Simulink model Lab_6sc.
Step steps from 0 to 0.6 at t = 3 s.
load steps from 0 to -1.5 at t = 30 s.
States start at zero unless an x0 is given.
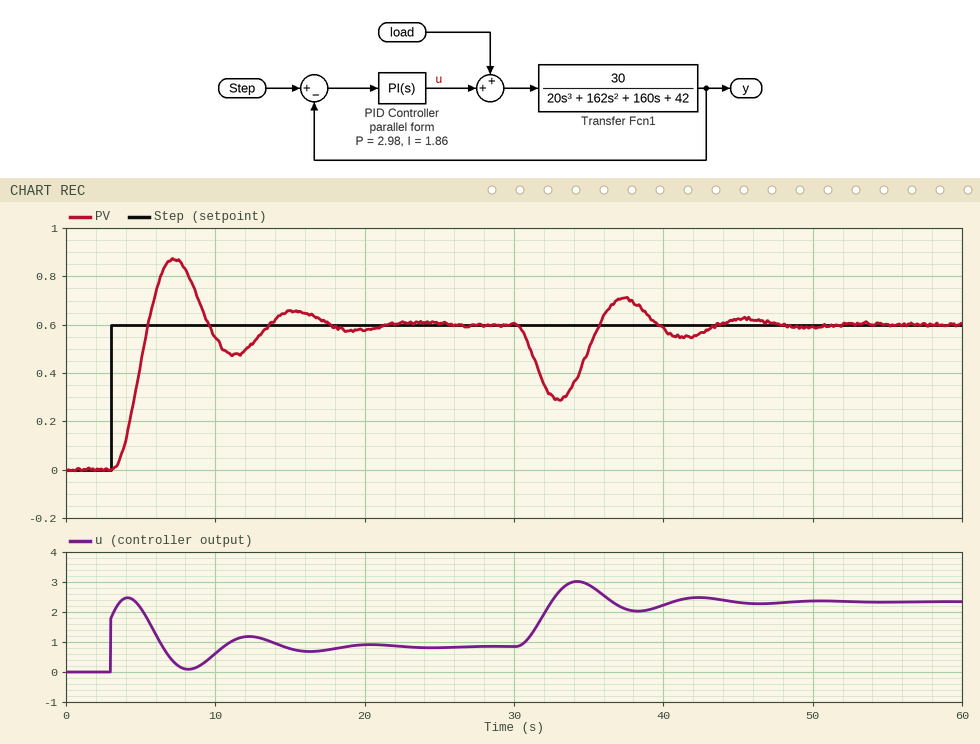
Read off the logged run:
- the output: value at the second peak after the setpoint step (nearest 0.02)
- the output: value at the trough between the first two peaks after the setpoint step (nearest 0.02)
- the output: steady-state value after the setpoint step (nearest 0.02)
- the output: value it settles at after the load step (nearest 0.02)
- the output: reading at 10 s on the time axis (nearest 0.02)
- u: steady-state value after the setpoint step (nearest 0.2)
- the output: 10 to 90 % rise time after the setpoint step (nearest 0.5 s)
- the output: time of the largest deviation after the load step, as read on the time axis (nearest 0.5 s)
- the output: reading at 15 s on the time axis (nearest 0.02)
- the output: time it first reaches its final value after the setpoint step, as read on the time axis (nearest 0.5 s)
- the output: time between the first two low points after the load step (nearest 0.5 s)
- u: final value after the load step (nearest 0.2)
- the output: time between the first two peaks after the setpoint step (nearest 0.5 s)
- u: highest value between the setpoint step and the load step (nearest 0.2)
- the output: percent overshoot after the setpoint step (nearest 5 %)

0.66
0.48
0.60
0.60
0.54
0.8
1.5 s
33.0 s
0.66
5.5 s
8.5 s
2.4
8.0 s
2.4
45 %
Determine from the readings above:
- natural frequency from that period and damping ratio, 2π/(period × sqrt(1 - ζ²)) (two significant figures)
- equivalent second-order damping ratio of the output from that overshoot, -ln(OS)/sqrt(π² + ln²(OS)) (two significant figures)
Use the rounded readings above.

0.81 rad/s
0.25
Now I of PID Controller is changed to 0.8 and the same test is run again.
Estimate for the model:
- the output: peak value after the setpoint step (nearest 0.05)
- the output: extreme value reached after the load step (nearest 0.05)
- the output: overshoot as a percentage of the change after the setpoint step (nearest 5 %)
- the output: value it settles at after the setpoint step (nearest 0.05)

0.65
0.25
10 %
0.60
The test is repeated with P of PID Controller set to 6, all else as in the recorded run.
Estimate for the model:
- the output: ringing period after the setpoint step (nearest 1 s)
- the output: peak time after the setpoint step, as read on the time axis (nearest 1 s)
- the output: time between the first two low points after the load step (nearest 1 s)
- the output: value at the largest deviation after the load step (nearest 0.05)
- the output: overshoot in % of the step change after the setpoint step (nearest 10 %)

6 s
6 s
6 s
0.35
40 %
